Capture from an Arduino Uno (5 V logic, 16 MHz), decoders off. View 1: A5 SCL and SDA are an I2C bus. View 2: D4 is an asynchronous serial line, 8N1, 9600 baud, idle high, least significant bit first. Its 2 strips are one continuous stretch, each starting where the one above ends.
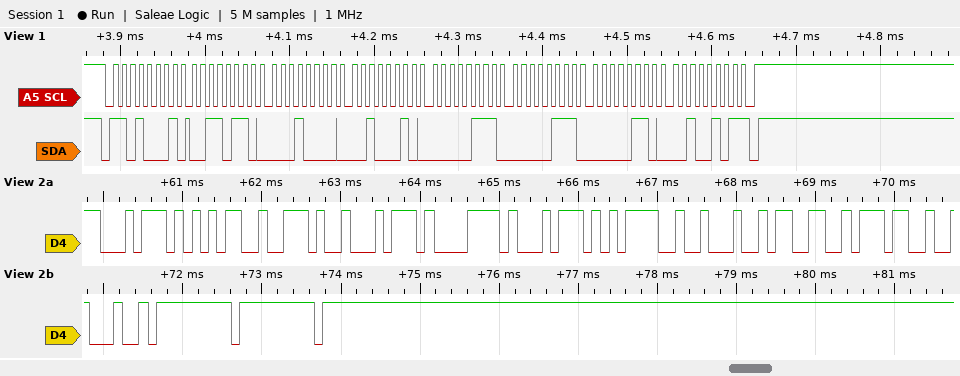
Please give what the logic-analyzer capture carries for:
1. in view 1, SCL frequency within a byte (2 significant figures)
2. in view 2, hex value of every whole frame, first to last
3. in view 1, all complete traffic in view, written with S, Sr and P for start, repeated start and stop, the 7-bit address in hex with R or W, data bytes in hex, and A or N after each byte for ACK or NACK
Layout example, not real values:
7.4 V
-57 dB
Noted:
100 kHz
74 35 2E 74 78 74 3D 22 33 37 22 FF FF FF
S 68R A 36 A 10 A 22 A 07 A 07 A 06 A 25 N P
